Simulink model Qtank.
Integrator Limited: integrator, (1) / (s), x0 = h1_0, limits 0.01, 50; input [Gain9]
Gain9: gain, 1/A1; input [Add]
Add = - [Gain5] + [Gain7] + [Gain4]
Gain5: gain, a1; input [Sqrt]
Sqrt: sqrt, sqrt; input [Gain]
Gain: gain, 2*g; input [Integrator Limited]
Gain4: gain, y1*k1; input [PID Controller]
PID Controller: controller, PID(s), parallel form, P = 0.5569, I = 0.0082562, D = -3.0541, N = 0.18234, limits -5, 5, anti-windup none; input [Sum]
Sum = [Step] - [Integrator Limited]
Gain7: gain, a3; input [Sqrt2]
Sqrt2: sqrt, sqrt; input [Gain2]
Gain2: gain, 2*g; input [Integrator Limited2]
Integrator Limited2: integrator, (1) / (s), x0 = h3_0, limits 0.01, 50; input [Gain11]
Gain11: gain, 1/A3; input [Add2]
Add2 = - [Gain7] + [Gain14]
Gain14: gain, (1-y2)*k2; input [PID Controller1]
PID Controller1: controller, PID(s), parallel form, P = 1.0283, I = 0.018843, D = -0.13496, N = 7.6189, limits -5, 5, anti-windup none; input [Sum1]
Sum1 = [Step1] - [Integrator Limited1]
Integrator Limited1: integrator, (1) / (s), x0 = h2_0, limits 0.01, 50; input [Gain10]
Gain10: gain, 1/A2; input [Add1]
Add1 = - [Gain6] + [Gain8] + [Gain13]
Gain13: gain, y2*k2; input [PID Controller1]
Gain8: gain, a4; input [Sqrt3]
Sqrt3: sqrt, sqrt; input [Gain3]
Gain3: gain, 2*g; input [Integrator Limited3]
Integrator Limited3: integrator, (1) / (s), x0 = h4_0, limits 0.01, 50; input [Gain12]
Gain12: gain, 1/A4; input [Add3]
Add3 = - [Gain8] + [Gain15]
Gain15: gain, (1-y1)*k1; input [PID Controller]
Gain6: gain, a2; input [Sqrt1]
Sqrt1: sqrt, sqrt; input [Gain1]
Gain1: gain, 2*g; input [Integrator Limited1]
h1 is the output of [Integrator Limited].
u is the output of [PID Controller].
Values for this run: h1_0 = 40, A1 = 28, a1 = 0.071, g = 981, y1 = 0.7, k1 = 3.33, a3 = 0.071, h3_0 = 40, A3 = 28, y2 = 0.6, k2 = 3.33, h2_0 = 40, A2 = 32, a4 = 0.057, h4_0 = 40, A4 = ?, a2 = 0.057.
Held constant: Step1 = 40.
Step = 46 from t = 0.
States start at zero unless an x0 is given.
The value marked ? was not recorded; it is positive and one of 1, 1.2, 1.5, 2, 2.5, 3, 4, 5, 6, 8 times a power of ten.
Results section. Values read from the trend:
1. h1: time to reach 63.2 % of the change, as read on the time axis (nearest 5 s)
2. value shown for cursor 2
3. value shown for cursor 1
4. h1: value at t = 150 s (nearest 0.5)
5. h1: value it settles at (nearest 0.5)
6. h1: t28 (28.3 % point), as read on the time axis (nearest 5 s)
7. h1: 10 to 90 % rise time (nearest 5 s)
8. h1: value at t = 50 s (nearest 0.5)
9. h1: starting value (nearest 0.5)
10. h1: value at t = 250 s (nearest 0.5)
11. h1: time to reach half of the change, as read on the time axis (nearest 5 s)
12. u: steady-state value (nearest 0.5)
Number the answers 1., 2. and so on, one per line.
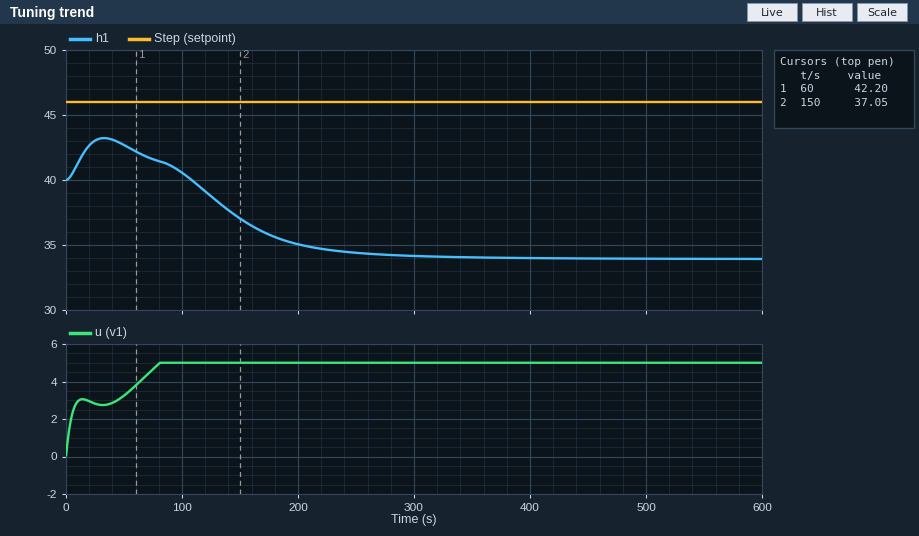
1. 165 s
2. 37.05
3. 42.20
4. 37.0
5. 34.0
6. 130 s
7. 120 s
8. 42.5
9. 40.0
10. 34.5
11. 150 s
12. 5.0
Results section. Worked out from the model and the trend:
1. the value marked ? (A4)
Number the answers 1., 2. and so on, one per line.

1. 30
